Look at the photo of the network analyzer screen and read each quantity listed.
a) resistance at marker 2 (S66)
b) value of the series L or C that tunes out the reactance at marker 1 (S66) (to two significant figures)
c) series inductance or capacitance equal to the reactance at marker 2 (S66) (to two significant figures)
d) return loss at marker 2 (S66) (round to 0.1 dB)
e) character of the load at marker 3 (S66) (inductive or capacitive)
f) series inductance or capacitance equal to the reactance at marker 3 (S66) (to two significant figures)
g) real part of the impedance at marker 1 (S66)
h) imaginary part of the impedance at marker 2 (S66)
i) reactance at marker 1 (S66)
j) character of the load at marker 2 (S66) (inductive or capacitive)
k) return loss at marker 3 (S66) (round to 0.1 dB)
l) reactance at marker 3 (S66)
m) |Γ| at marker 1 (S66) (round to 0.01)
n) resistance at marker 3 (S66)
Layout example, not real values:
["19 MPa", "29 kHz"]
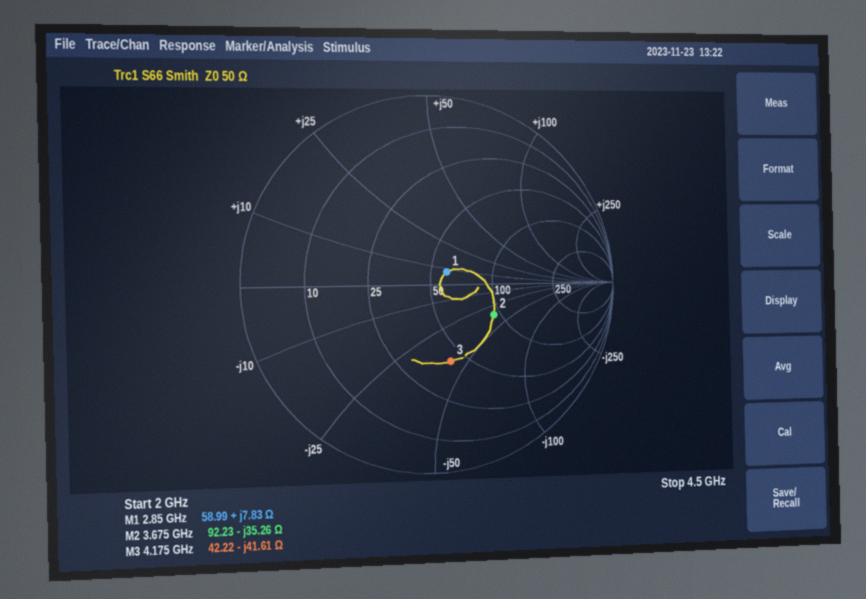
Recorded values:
["92.23 Ω", "7.1 pF", "1.2 pF", "8.5 dB", "capacitive", "920 fF", "58.99 Ω", "-35.26 Ω", "+7.83 Ω", "capacitive", "7.6 dB", "-41.61 Ω", "0.11", "42.22 Ω"]
